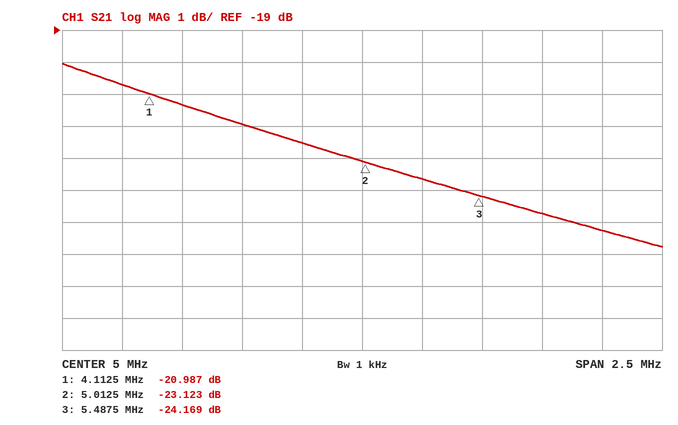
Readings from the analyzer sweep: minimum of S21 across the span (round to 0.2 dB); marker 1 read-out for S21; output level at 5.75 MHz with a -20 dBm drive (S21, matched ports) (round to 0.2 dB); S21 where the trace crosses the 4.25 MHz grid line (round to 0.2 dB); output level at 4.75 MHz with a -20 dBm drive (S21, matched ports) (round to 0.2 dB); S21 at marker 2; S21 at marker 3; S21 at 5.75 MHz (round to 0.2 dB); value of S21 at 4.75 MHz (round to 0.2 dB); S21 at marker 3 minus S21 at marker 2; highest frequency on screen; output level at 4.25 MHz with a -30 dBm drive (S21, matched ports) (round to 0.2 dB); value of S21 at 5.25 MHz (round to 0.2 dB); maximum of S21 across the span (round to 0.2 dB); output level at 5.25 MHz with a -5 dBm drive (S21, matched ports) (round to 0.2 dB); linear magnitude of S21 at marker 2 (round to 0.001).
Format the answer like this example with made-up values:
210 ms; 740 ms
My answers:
-25.8 dB; -20.987 dB; -44.8 dBm; -21.4 dB; -42.6 dBm; -23.123 dB; -24.169 dB; -24.8 dB; -22.6 dB; -1.046 dB; 6.25 MHz; -51.4 dBm; -23.6 dB; -20.0 dB; -28.6 dBm; 0.070
